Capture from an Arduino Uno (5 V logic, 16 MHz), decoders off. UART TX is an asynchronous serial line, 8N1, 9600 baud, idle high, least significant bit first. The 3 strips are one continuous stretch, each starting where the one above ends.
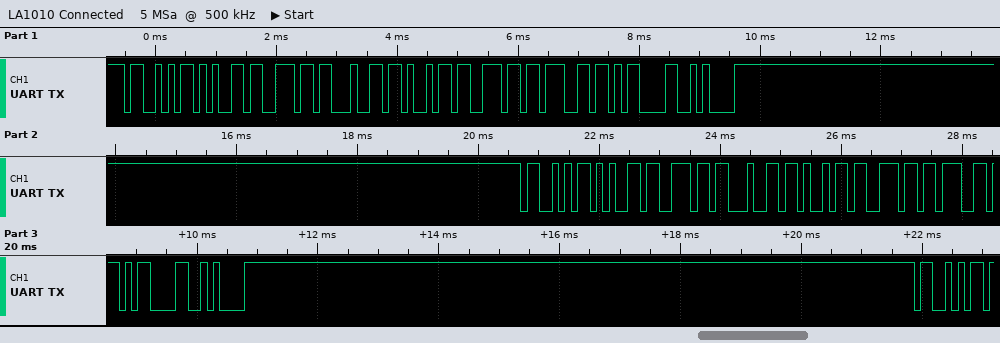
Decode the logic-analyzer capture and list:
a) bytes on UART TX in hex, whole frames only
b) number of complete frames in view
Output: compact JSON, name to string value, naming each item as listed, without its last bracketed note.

{"bytes on UART TX in hex, whole frames only": "0x53 0x65 0x6E 0x64 0x69 0x6E 0x67 0x0D 0x0A 0x53 0x65 0x6E 0x64 0x69 0x6E 0x67 0x0D 0x0A 0x53", "number of complete frames in view": "19"}
